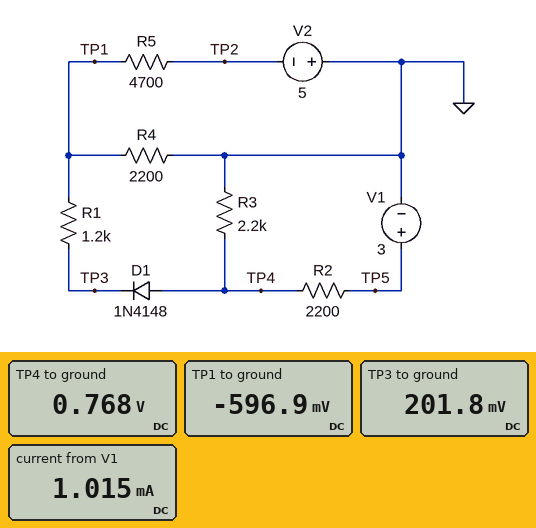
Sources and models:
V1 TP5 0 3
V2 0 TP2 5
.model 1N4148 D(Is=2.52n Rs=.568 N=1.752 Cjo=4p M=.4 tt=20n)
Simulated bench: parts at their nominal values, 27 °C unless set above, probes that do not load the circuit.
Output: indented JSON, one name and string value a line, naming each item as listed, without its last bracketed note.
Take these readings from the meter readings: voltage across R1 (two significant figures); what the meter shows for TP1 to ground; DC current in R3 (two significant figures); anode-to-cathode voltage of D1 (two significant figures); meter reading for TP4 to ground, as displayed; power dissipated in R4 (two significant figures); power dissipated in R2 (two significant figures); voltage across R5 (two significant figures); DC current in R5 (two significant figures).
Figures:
{
  "voltage across R1": "800 mV",
  "what the meter shows for TP1 to ground": "-596.9 mV",
  "DC current in R3": "350 µA",
  "anode-to-cathode voltage of D1": "570 mV",
  "meter reading for TP4 to ground, as displayed": "0.768 V",
  "power dissipated in R4": "160 µW",
  "power dissipated in R2": "2.3 mW",
  "voltage across R5": "4.4 V",
  "DC current in R5": "940 µA"
}
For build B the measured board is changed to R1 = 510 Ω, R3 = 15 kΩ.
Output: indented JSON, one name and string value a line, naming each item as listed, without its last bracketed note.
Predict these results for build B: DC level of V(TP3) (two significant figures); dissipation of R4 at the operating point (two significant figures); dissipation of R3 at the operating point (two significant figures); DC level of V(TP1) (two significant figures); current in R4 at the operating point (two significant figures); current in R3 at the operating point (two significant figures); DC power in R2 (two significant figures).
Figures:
{
  "DC level of V(TP3)": "260 mV",
  "dissipation of R4 at the operating point": "20 µW",
  "dissipation of R3 at the operating point": "47 µW",
  "DC level of V(TP1)": "-210 mV",
  "current in R4 at the operating point": "95 µA",
  "current in R3 at the operating point": "56 µA",
  "DC power in R2": "2.1 mW"
}
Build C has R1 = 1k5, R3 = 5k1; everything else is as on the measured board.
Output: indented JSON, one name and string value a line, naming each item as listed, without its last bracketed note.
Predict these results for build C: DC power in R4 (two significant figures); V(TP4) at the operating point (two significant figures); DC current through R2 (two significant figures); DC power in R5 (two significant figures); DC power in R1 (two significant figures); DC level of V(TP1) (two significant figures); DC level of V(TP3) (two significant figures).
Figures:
{
  "DC power in R4": "140 µW",
  "V(TP4) at the operating point": "1.0 V",
  "DC current through R2": "890 µA",
  "DC power in R5": "4.2 mW",
  "DC power in R1": "710 µW",
  "DC level of V(TP1)": "-560 mV",
  "DC level of V(TP3)": "470 mV"
}
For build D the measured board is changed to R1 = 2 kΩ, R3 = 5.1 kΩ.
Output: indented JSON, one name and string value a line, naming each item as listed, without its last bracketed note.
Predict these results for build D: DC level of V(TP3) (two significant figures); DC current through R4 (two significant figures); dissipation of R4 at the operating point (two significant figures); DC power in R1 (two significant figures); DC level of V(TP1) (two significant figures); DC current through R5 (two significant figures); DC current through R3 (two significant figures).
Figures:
{
  "DC level of V(TP3)": "580 mV",
  "DC current through R4": "300 µA",
  "dissipation of R4 at the operating point": "200 µW",
  "DC power in R1": "770 µW",
  "DC level of V(TP1)": "-660 mV",
  "DC current through R5": "920 µA",
  "DC current through R3": "220 µA"
}
